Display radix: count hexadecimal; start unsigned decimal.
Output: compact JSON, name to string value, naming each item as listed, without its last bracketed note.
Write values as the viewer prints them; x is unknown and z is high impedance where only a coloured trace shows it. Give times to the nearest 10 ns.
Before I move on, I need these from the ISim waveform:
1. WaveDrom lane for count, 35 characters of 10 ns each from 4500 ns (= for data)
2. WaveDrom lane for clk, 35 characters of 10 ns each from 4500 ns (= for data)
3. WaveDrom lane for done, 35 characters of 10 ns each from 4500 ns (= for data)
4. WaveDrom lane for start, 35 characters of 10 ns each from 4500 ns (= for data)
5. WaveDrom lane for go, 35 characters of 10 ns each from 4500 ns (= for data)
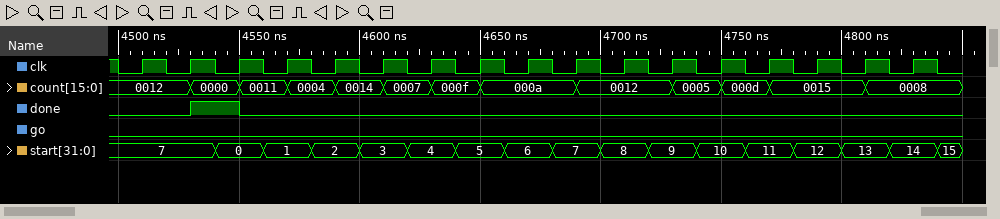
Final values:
{"WaveDrom lane for count, 35 characters of 10 ns each from 4500 ns": "{name: 'count', wave: '=..=.=.=.=.=.=.=...=...=.=.=...=...', data: '0012 0000 0011 0004 0014 0007 000f 000a 0012 0005 000d 0015 0008'}", "WaveDrom lane for clk, 35 characters of 10 ns each from 4500 ns": "{name: 'clk', wave: '01010101010101010101010101010101010'}", "WaveDrom lane for done, 35 characters of 10 ns each from 4500 ns": "{name: 'done', wave: '0..1.0.............................'}", "WaveDrom lane for start, 35 characters of 10 ns each from 4500 ns": "{name: 'start', wave: '=...=.=.=.=.=.=.=.=.=.=.=.=.=.=.=.=', data: '7 0 1 2 3 4 5 6 7 8 9 10 11 12 13 14 15'}", "WaveDrom lane for go, 35 characters of 10 ns each from 4500 ns": "{name: 'go', wave: '0..................................'}"}
